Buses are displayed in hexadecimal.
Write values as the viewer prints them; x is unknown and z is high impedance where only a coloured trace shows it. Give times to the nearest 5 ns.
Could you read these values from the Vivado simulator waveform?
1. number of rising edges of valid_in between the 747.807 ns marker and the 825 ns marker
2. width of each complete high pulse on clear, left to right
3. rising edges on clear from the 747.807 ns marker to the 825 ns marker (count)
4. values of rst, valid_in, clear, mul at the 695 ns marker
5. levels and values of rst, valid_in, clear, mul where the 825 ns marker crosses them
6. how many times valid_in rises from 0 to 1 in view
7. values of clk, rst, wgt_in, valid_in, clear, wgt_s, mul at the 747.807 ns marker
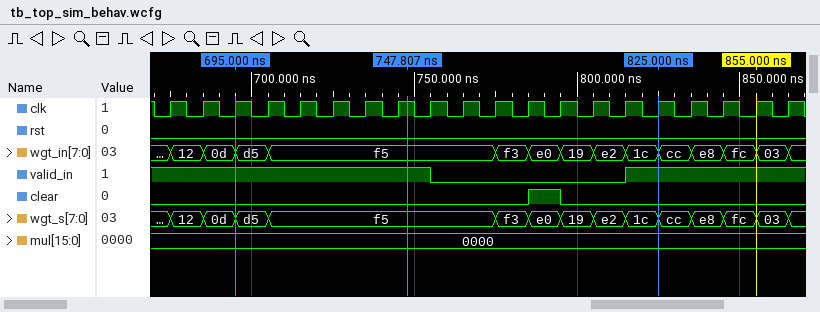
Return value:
1
10 ns
1
rst=0, valid_in=1, clear=0, mul=0000
rst=0, valid_in=1, clear=0, mul=0000
1
clk=1, rst=0, wgt_in=f5, valid_in=1, clear=0, wgt_s=f5, mul=0000
